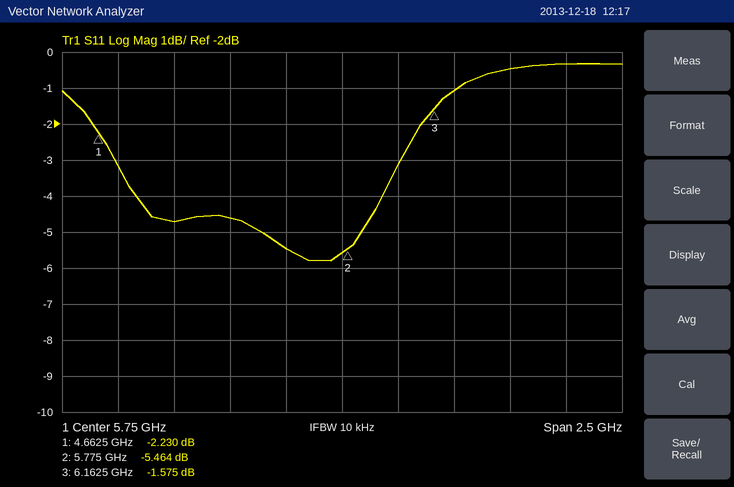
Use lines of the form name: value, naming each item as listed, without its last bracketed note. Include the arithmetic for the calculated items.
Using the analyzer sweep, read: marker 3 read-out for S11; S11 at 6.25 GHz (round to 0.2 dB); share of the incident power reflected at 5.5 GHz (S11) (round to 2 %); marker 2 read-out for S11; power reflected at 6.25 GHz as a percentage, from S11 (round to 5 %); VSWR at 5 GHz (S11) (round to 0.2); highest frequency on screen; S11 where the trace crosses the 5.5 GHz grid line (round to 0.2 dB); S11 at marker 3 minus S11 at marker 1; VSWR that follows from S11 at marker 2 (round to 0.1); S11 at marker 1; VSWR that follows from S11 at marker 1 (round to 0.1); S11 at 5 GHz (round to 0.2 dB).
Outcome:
marker 3 read-out for S11: -1.575 dB
S11 at 6.25 GHz: -1.0 dB
share of the incident power reflected at 5.5 GHz (S11): 10^(-5.4/10) ≈ 28.8 %, so 28 % to the nearest 2 %
marker 2 read-out for S11: -5.464 dB
power reflected at 6.25 GHz as a percentage, from S11: 10^(-1/10) ≈ 79.4 %, so 80 % to the nearest 5 %
VSWR at 5 GHz (S11): |Γ| = 10^(-4.8/20) = 0.5754; VSWR = (1 + 0.5754)/(1 − 0.5754) ≈ 3.71, so 3.8 to the nearest 0.2
highest frequency on screen: 7 GHz
S11 where the trace crosses the 5.5 GHz grid line: -5.4 dB
S11 at marker 3 minus S11 at marker 1: -1.575 − (-2.23) = 0.655 dB
VSWR that follows from S11 at marker 2: (1 + 0.5331)/(1 − 0.5331) ≈ 3.3
S11 at marker 1: -2.230 dB
VSWR that follows from S11 at marker 1: (1 + 0.7736)/(1 − 0.7736) ≈ 7.8
S11 at 5 GHz: -4.8 dB
